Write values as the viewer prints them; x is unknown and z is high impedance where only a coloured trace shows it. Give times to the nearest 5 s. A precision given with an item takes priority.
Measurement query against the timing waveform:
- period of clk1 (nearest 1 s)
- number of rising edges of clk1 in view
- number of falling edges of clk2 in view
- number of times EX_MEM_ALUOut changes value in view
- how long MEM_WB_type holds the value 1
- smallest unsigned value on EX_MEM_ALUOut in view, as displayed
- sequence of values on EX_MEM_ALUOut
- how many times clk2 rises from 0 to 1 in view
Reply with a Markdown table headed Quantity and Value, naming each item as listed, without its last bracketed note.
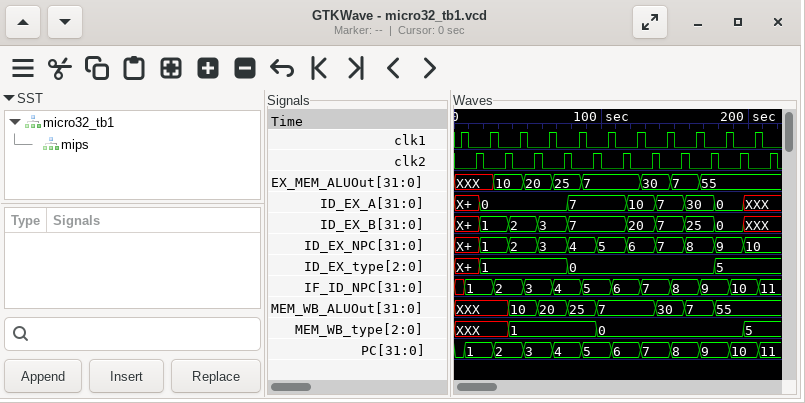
| Quantity | Value |
|---|---|
| period of clk1 | 20 s |
| number of rising edges of clk1 in view | 11 |
| number of falling edges of clk2 in view | 11 |
| number of times EX_MEM_ALUOut changes value in view | 7 |
| how long MEM_WB_type holds the value 1 | 60 s |
| smallest unsigned value on EX_MEM_ALUOut in view, as displayed | 7 |
| sequence of values on EX_MEM_ALUOut | XXX, 10, 20, 25, 7, 30, 7, 55 |
| how many times clk2 rises from 0 to 1 in view | 11 |
